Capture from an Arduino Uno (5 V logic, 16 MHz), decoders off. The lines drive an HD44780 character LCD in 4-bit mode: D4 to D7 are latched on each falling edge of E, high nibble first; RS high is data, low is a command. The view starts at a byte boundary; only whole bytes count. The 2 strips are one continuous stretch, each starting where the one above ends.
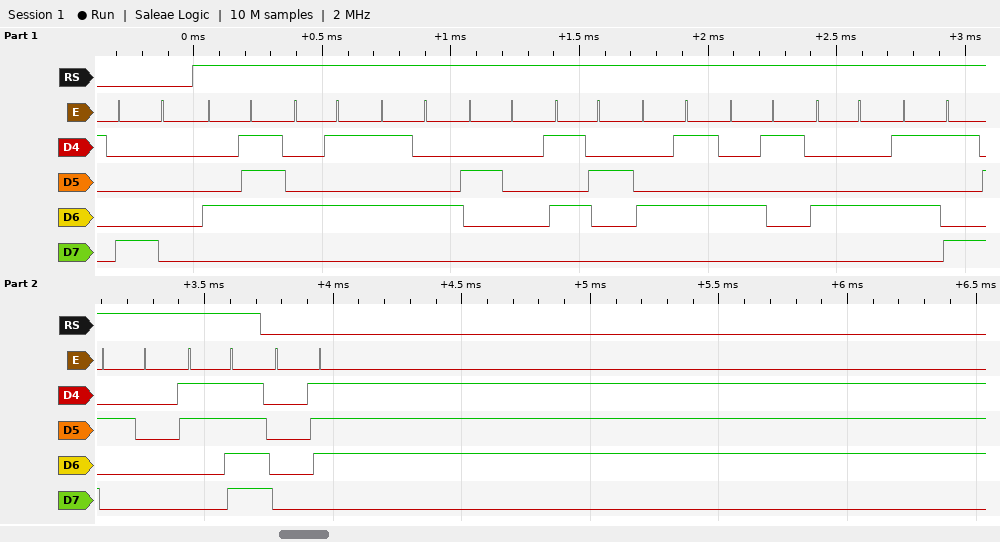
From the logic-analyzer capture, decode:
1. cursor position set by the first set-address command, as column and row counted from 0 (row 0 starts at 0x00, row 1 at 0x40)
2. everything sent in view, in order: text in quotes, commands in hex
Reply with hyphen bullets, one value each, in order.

- column 0, row 0
- 0x80 "GET READY ?" 0x07
